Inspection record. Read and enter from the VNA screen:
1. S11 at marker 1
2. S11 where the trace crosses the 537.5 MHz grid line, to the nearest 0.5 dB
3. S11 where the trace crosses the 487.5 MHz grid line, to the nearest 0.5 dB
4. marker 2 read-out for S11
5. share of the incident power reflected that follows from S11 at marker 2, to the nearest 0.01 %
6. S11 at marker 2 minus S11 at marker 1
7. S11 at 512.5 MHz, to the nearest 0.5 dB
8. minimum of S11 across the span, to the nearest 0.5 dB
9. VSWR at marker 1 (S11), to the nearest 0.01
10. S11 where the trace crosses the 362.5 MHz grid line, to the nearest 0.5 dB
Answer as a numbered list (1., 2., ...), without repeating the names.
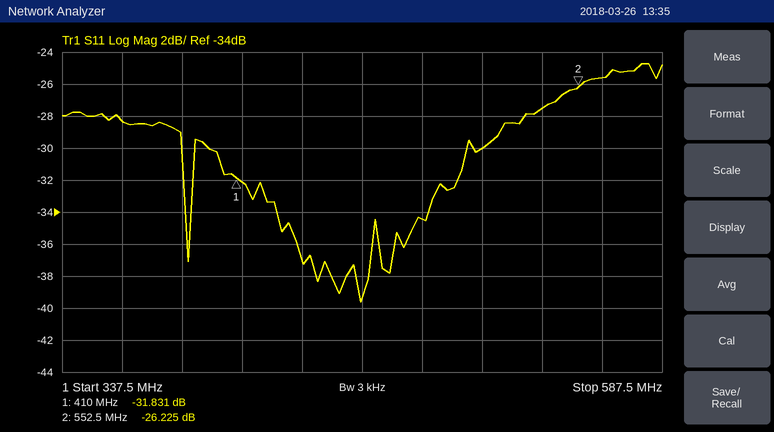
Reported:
1. -31.831 dB
2. -27.5 dB
3. -34.5 dB
4. -26.225 dB
5. 0.24 %
6. 5.606 dB
7. -30.0 dB
8. -39.5 dB
9. 1.05
10. -28.5 dB
